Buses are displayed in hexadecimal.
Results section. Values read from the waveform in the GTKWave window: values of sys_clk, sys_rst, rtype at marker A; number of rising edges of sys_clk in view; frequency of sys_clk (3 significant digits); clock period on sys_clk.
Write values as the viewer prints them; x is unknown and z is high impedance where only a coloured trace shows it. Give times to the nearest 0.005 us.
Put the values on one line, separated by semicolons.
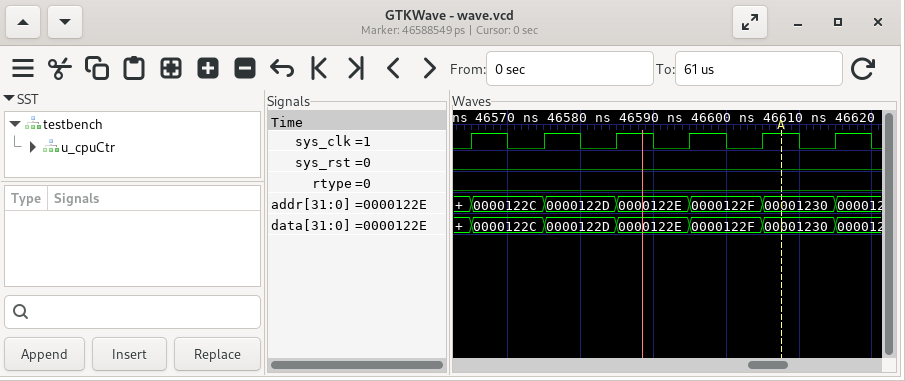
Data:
sys_clk=1, sys_rst=0, rtype=0; 6; 100 MHz; 0.01 us
